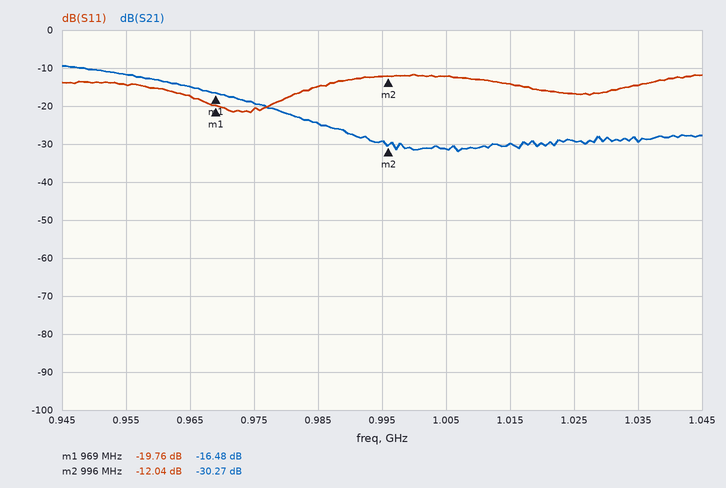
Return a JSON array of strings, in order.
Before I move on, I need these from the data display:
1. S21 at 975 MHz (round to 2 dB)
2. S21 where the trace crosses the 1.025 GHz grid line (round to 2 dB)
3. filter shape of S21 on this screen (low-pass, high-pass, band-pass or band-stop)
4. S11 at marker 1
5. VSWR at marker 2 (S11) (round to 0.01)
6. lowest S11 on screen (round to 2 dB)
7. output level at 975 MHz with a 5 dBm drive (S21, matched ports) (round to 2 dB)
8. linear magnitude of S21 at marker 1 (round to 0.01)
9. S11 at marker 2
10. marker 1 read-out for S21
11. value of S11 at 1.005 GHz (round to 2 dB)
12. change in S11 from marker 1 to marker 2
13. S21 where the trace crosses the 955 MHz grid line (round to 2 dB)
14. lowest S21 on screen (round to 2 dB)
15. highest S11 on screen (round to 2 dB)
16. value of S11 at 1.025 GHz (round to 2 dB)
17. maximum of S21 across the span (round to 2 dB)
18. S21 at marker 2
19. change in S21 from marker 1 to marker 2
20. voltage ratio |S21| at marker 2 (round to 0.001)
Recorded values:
["-20 dB", "-30 dB", "low-pass", "-19.76 dB", "1.67", "-22 dB", "-14 dBm", "0.15", "-12.04 dB", "-16.48 dB", "-12 dB", "7.72 dB", "-12 dB", "-32 dB", "-12 dB", "-16 dB", "-10 dB", "-30.27 dB", "-13.79 dB", "0.031"]
